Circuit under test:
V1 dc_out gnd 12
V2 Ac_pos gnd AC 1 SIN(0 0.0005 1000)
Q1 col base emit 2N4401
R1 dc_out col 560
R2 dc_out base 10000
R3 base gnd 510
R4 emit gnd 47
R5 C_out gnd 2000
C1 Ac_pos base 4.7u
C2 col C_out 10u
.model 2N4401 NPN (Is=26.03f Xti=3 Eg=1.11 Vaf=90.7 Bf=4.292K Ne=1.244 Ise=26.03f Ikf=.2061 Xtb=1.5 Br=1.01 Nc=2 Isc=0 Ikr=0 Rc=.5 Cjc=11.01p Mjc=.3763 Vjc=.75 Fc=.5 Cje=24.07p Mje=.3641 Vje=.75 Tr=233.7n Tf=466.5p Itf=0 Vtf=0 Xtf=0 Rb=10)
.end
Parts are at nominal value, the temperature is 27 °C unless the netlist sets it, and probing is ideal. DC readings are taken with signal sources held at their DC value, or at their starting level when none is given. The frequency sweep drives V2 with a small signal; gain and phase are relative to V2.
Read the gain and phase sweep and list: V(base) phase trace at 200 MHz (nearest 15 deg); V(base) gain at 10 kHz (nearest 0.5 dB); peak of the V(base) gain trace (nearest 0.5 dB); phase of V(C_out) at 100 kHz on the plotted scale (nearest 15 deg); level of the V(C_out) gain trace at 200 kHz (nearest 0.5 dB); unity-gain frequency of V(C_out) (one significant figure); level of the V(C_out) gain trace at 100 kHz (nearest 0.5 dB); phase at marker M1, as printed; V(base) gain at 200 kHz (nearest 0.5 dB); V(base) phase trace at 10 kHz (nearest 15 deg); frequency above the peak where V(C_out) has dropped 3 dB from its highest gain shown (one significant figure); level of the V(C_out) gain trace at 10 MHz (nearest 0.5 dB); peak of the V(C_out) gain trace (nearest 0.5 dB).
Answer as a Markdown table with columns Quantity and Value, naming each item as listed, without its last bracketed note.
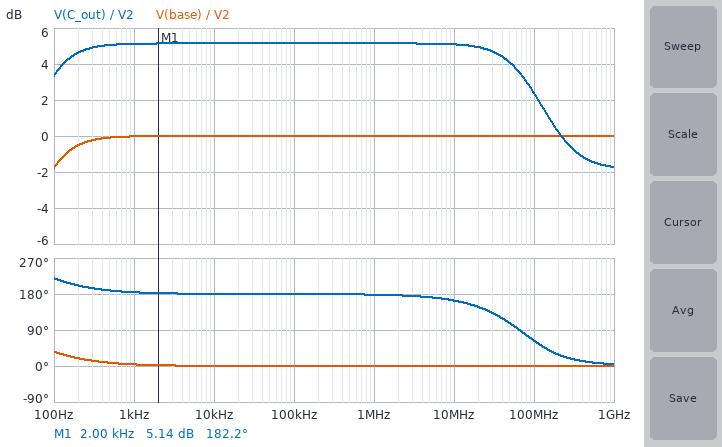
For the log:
| Quantity | Value |
|---|---|
| V(base) phase trace at 200 MHz | 0 deg |
| V(base) gain at 10 kHz | 0 dB |
| peak of the V(base) gain trace | 0 dB |
| phase of V(C_out) at 100 kHz on the plotted scale | 180 deg |
| level of the V(C_out) gain trace at 200 kHz | 5.0 dB |
| unity-gain frequency of V(C_out) | 200 MHz |
| level of the V(C_out) gain trace at 100 kHz | 5.0 dB |
| phase at marker M1, as printed | 182.2 deg |
| V(base) gain at 200 kHz | 0 dB |
| V(base) phase trace at 10 kHz | 0 deg |
| frequency above the peak where V(C_out) has dropped 3 dB from its highest gain shown | 100 MHz |
| level of the V(C_out) gain trace at 10 MHz | 5.0 dB |
| peak of the V(C_out) gain trace | 5.0 dB |
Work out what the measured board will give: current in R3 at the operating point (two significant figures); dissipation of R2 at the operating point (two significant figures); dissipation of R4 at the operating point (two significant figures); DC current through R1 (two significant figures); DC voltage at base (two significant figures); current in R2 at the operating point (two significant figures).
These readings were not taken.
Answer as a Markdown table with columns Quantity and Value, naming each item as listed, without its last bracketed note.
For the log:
| Quantity | Value |
|---|---|
| current in R3 at the operating point | 1.1 mA |
| dissipation of R2 at the operating point | 13 mW |
| dissipation of R4 at the operating point | 850 nW |
| DC current through R1 | 130 µA |
| DC voltage at base | 580 mV |
| current in R2 at the operating point | 1.1 mA |
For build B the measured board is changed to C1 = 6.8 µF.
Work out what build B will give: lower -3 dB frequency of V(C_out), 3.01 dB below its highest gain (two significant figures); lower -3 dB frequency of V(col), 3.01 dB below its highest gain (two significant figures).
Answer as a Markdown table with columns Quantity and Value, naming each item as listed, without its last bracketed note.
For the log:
| Quantity | Value |
|---|---|
| lower -3 dB frequency of V(C_out), 3.01 dB below its highest gain | 50 Hz |
| lower -3 dB frequency of V(col), 3.01 dB below its highest gain | 49 Hz |
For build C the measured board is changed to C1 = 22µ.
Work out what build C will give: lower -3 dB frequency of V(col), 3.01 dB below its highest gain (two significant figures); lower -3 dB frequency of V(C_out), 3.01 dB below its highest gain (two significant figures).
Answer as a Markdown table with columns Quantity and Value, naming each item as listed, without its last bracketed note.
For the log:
| Quantity | Value |
|---|---|
| lower -3 dB frequency of V(col), 3.01 dB below its highest gain | 14 Hz |
| lower -3 dB frequency of V(C_out), 3.01 dB below its highest gain | 17 Hz |
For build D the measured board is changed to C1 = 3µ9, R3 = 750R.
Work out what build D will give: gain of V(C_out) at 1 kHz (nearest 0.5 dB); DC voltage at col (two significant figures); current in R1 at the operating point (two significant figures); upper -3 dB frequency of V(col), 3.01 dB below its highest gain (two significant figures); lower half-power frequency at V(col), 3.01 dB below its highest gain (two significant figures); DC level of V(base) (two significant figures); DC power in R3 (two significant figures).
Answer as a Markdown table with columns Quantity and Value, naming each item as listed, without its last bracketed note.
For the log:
| Quantity | Value |
|---|---|
| gain of V(C_out) at 1 kHz | 18.0 dB |
| DC voltage at col | 10 V |
| current in R1 at the operating point | 3.4 mA |
| upper -3 dB frequency of V(col), 3.01 dB below its highest gain | 67 MHz |
| lower half-power frequency at V(col), 3.01 dB below its highest gain | 62 Hz |
| DC level of V(base) | 820 mV |
| DC power in R3 | 900 µW |
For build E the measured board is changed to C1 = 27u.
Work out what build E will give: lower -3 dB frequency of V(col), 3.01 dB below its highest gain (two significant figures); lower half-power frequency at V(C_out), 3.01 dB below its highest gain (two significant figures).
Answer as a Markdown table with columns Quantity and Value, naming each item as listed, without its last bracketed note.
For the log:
| Quantity | Value |
|---|---|
| lower -3 dB frequency of V(col), 3.01 dB below its highest gain | 11 Hz |
| lower half-power frequency at V(C_out), 3.01 dB below its highest gain | 15 Hz |
